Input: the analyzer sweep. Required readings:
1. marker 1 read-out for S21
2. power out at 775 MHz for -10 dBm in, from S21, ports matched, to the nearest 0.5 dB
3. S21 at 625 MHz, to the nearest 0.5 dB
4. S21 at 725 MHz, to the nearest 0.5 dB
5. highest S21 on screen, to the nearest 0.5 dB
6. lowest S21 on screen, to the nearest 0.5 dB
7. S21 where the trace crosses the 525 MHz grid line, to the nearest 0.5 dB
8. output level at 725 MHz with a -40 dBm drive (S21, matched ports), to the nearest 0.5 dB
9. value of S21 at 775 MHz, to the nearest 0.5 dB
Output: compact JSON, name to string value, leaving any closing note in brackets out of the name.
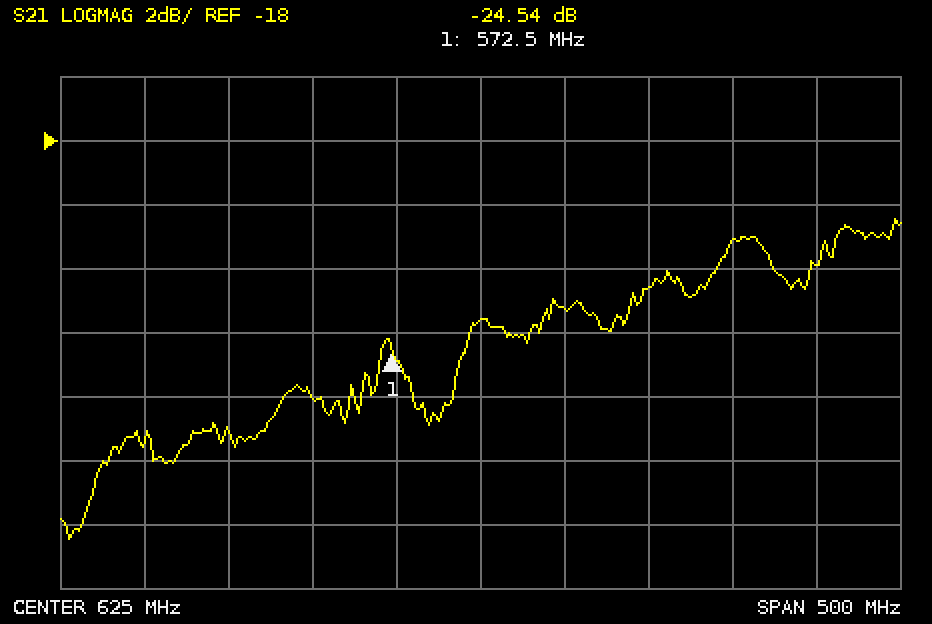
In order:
{"marker 1 read-out for S21": "-24.54 dB", "power out at 775 MHz for -10 dBm in, from S21, ports matched, to the nearest 0.5 dB": "-31.0 dBm", "S21 at 625 MHz, to the nearest 0.5 dB": "-23.5 dB", "S21 at 725 MHz, to the nearest 0.5 dB": "-22.5 dB", "highest S21 on screen, to the nearest 0.5 dB": "-20.5 dB", "lowest S21 on screen, to the nearest 0.5 dB": "-30.5 dB", "S21 where the trace crosses the 525 MHz grid line, to the nearest 0.5 dB": "-26.0 dB", "output level at 725 MHz with a -40 dBm drive (S21, matched ports), to the nearest 0.5 dB": "-62.5 dBm", "value of S21 at 775 MHz, to the nearest 0.5 dB": "-21.0 dB"}
